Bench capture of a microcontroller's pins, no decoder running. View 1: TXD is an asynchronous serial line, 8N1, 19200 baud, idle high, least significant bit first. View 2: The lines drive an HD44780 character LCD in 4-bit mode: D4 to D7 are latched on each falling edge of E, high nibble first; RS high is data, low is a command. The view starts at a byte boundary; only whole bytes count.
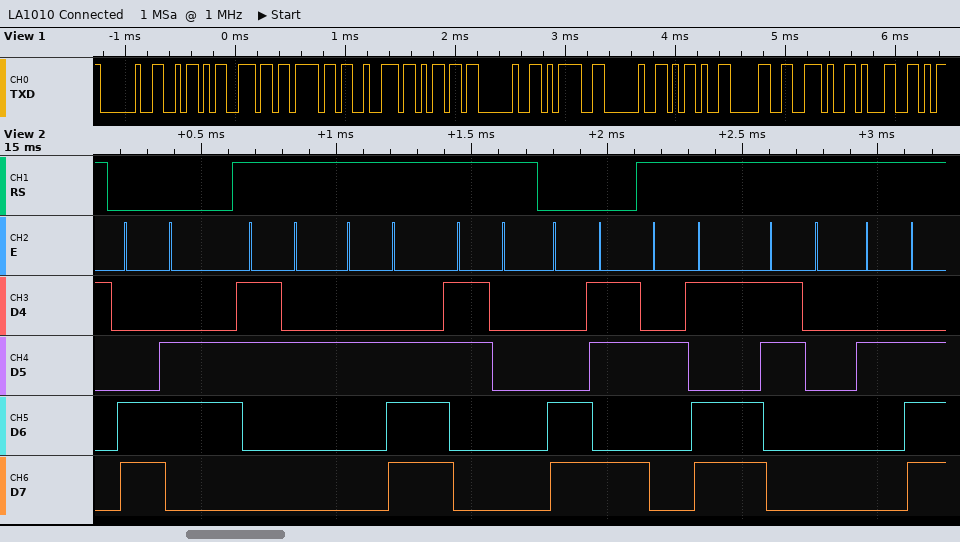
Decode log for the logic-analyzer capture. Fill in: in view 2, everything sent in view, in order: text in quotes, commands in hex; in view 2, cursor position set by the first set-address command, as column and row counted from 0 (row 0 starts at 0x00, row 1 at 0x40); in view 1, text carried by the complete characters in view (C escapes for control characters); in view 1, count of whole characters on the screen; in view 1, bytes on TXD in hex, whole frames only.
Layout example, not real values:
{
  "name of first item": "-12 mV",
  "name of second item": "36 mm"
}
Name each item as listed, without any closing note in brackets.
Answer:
{
  "in view 2, everything sent in view, in order: text in quotes, commands in hex": "0xC6 \"2.0\" 0xCB \"-0.\"",
  "in view 2, cursor position set by the first set-address command, as column and row counted from 0": "column 6, row 1",
  "in view 1, text carried by the complete characters in view": "\" Znorm = -0.1\"",
  "in view 1, count of whole characters on the screen": "13",
  "in view 1, bytes on TXD in hex, whole frames only": "0x20 0x5A 0x6E 0x6F 0x72 0x6D 0x20 0x3D 0x20 0x2D 0x30 0x2E 0x31"
}
